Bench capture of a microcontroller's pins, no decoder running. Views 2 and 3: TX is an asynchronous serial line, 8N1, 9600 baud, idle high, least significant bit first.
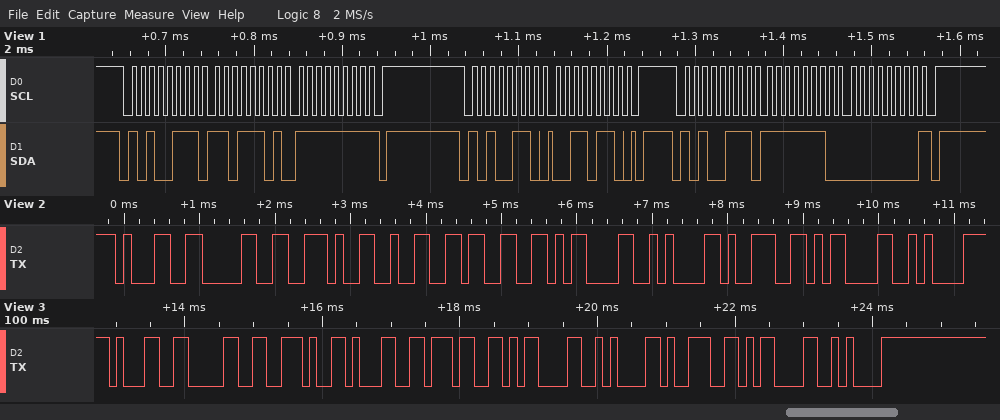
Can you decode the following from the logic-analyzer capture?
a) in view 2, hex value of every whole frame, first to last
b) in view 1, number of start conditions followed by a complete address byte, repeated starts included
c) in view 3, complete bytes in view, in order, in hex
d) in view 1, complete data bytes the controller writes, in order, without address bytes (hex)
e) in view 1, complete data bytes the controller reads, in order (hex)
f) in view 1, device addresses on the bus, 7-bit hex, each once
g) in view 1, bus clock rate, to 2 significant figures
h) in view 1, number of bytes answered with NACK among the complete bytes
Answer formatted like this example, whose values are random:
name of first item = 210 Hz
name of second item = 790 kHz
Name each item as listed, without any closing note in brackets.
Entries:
in view 2, hex value of every whole frame, first to last = 31 30 2E 32 33 0D 0A 39 0D 0A
in view 1, number of start conditions followed by a complete address byte, repeated starts included = 3
in view 3, complete bytes in view, in order, in hex = 31 30 2E 31 37 0D 0A 39 0D 0A
in view 1, complete data bytes the controller writes, in order, without address bytes = 36
in view 1, complete data bytes the controller reads, in order = DD FF FE 00
in view 1, device addresses on the bus, 7-bit hex, each once = 0x53
in view 1, bus clock rate, to 2 significant figures = 100 kHz
in view 1, number of bytes answered with NACK among the complete bytes = 2
